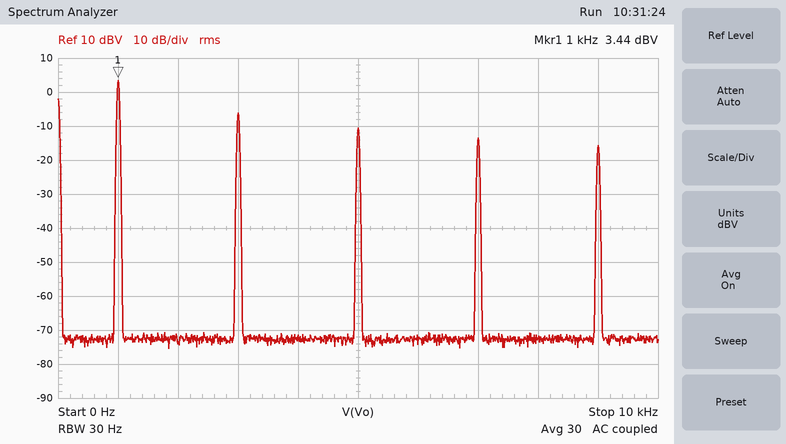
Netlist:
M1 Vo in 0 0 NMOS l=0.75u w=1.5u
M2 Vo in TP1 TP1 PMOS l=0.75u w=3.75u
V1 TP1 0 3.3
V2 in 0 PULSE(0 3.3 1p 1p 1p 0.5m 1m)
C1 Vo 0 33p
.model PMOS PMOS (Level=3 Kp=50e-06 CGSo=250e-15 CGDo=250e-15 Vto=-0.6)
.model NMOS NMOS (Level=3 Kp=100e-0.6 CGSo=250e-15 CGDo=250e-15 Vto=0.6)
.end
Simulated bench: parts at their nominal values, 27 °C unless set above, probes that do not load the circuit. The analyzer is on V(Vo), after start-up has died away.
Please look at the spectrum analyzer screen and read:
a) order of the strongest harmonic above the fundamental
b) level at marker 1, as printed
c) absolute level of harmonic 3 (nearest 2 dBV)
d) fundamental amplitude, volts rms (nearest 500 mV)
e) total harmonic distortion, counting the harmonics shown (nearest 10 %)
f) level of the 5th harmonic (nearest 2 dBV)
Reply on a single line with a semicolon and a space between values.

3; 3.44 dBV; -6 dBV; 1.5 V; 40 %; -10 dBV
